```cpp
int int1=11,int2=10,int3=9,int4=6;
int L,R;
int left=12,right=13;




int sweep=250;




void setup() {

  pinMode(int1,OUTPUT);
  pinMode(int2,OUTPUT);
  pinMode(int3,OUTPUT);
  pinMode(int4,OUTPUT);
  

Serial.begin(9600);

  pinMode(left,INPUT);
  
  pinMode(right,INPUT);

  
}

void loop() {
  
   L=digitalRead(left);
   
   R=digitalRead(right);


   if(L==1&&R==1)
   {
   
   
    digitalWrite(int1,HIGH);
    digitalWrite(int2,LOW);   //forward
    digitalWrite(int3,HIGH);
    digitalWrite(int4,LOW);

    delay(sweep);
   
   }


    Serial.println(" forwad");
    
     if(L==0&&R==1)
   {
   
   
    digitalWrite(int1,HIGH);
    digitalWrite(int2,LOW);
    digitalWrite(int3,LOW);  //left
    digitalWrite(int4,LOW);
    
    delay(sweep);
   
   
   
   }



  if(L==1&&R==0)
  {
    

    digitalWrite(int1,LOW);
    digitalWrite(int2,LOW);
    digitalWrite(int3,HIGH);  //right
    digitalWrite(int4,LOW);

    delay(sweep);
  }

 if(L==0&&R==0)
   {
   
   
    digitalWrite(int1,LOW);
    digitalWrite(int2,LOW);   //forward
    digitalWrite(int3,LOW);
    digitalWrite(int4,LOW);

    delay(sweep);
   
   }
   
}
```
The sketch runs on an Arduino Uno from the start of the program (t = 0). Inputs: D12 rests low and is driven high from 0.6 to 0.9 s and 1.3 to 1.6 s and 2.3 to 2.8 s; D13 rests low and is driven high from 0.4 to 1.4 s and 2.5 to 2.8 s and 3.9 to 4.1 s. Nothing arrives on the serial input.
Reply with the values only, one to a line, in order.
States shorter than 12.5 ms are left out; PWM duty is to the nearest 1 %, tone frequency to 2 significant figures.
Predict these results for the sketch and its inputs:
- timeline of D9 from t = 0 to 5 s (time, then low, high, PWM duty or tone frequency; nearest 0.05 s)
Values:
0 s low; 0.75 s high; 1 s low; 1.5 s high; 1.75 s low; 2.5 s high; 3 s low
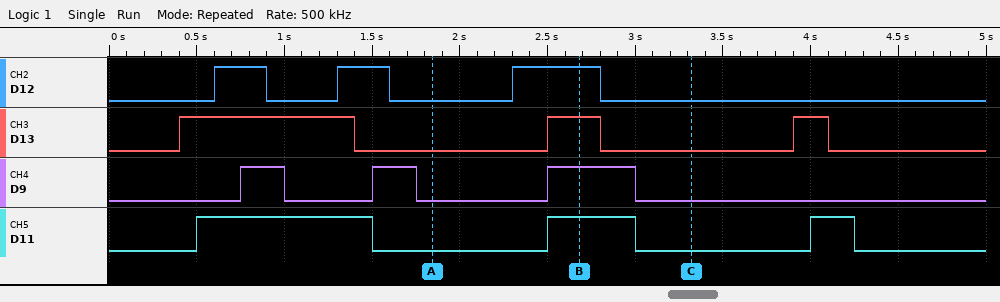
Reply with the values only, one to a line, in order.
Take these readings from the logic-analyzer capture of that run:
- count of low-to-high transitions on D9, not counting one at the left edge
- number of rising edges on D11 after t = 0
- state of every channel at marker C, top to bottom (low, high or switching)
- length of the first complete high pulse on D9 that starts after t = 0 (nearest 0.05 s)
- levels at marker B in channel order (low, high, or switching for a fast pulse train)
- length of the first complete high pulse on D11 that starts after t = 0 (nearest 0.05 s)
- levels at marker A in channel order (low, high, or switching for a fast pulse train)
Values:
3
3
D12 low, D13 low, D9 low, D11 low
0.25 s
D12 high, D13 high, D9 high, D11 high
1.00 s
D12 low, D13 low, D9 low, D11 low
